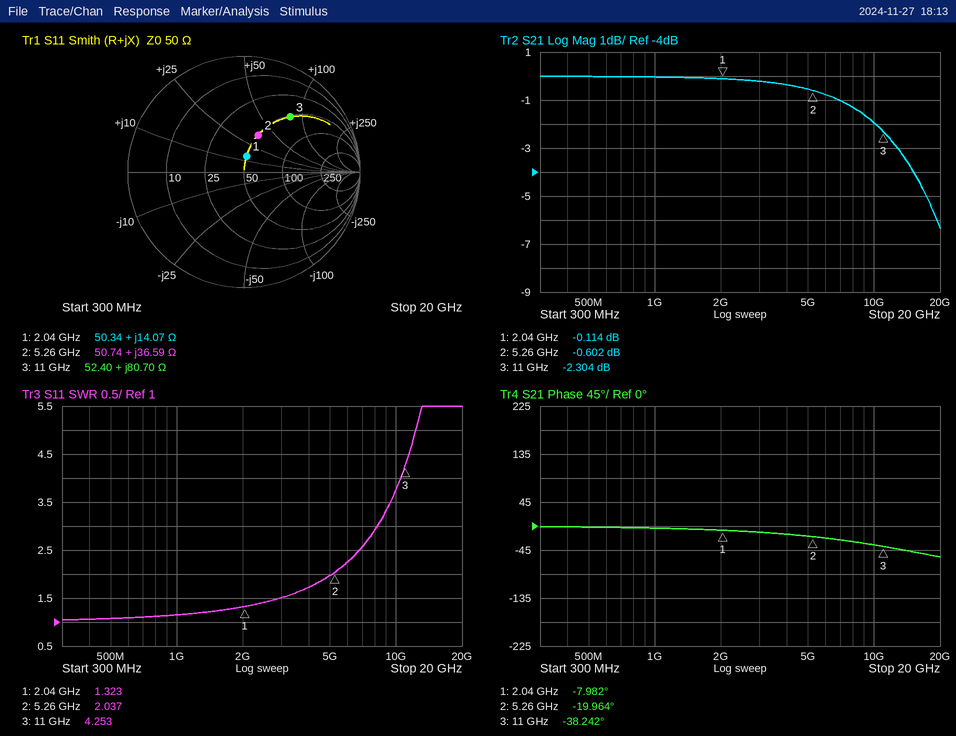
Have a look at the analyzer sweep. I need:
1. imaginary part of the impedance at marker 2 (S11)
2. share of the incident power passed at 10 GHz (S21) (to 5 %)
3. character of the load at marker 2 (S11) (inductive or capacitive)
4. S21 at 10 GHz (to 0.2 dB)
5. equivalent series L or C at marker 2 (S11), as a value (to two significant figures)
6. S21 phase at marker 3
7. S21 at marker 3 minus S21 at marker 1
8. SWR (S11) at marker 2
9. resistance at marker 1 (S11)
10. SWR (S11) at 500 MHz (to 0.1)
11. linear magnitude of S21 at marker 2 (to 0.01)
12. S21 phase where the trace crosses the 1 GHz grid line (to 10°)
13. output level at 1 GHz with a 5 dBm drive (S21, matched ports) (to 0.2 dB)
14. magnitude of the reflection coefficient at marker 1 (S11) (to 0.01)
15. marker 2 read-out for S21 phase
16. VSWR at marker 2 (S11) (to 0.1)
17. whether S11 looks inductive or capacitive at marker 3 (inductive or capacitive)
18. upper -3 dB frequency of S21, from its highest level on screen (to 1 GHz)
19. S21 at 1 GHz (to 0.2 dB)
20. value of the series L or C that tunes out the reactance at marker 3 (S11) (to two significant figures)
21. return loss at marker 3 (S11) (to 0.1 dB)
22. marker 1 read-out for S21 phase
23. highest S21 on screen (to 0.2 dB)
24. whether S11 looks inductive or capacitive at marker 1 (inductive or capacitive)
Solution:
+36.59 Ω
65 %
inductive
-2.0 dB
1.1 nH
-38.242°
-2.190 dB
2.037
50.34 Ω
1.1
0.93
0°
5.0 dBm
0.14
-19.964°
2.0
inductive
13 GHz
0.0 dB
180 fF
4.2 dB
-7.982°
0.0 dB
inductive
